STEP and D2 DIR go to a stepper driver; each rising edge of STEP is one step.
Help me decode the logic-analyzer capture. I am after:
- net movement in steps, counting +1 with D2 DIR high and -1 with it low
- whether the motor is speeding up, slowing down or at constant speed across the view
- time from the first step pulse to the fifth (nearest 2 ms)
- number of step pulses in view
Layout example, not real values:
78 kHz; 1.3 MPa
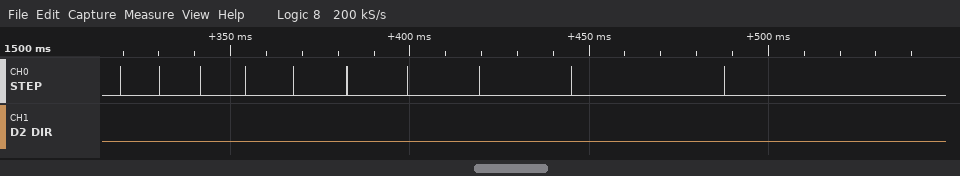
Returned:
-10; slowing down; 48 ms; 10
